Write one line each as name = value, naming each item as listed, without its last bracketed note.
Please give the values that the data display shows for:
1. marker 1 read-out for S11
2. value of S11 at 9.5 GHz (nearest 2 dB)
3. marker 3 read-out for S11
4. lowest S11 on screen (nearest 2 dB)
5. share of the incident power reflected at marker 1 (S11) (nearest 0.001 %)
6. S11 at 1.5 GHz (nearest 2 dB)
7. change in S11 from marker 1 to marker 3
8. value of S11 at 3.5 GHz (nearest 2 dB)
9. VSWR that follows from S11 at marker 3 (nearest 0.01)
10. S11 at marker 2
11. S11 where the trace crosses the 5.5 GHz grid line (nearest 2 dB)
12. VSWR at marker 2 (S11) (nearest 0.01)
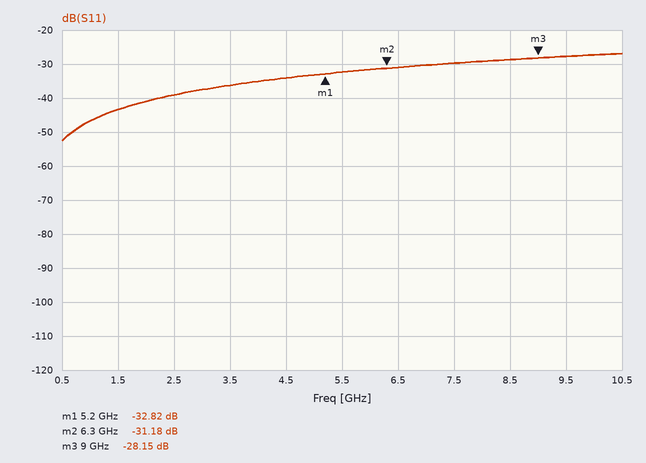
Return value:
marker 1 read-out for S11 = -32.82 dB
value of S11 at 9.5 GHz = -28 dB
marker 3 read-out for S11 = -28.15 dB
lowest S11 on screen = -52 dB
share of the incident power reflected at marker 1 (S11) = 0.052 %
S11 at 1.5 GHz = -44 dB
change in S11 from marker 1 to marker 3 = 4.67 dB
value of S11 at 3.5 GHz = -36 dB
VSWR that follows from S11 at marker 3 = 1.08
S11 at marker 2 = -31.18 dB
S11 where the trace crosses the 5.5 GHz grid line = -32 dB
VSWR at marker 2 (S11) = 1.06
